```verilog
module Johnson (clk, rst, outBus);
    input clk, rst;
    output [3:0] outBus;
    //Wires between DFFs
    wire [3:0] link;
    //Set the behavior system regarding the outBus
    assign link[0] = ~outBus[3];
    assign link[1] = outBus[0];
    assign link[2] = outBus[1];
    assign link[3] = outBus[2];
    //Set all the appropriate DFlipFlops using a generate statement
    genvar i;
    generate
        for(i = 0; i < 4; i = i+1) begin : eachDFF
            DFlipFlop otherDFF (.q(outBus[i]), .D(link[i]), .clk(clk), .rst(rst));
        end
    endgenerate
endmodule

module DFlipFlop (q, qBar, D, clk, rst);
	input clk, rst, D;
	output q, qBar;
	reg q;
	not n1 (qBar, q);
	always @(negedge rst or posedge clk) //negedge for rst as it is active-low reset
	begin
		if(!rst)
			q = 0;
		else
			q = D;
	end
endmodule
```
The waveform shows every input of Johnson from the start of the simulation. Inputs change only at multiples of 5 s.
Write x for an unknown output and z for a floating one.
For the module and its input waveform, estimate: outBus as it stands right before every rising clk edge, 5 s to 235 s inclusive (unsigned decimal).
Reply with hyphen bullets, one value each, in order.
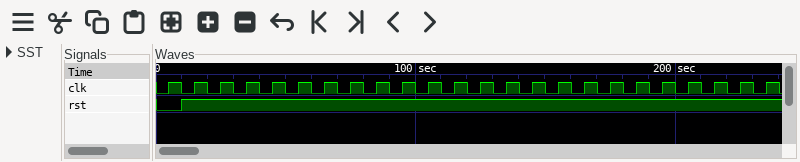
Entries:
- 0, 0, 1, 3, 7, 15, 14, 12, 8, 0, 1, 3, 7, 15, 14, 12, 8, 0, 1, 3, 7, 15, 14, 12
